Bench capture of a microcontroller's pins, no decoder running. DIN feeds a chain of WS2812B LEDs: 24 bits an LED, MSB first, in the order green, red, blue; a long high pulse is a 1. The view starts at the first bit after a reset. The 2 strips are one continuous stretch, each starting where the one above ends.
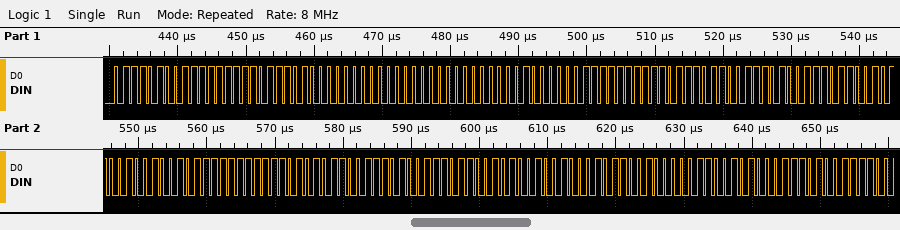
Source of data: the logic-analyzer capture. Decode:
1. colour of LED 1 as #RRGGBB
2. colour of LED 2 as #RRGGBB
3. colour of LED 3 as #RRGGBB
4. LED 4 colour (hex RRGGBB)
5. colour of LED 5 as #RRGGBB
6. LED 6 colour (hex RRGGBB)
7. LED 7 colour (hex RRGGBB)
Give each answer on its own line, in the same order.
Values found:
#FF74BA
#000000
#FF81BB
#763A52
#FF4BAB
#763A52
#904565
